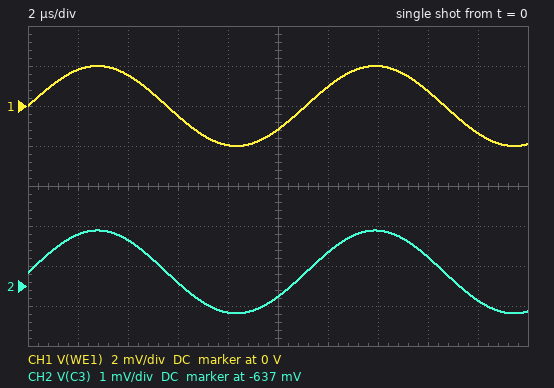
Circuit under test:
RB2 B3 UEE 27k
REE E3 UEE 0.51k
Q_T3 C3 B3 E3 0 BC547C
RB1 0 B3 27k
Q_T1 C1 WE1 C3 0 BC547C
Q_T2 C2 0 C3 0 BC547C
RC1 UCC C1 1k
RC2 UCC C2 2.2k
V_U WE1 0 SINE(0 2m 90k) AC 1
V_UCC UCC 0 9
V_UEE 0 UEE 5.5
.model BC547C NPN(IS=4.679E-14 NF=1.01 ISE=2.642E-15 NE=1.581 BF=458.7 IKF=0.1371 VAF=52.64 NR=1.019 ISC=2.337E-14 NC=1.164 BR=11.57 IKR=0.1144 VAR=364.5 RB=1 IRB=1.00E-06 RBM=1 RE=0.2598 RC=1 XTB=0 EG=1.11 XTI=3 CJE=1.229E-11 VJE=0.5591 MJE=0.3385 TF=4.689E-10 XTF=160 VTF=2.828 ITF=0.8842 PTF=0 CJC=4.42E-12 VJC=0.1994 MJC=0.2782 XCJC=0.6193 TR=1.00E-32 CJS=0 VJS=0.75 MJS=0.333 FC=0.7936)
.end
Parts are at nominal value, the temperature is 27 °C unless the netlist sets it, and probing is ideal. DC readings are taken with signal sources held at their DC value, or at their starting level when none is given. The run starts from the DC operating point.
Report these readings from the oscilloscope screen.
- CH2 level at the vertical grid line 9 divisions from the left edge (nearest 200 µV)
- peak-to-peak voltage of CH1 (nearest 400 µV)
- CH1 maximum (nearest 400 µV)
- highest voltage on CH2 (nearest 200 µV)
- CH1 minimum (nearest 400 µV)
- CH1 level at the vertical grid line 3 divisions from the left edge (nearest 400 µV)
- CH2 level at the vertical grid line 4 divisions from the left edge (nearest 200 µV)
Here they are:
-637.4 mV
4.0 mV
2.0 mV
-635.6 mV
-2.0 mV
-400 µV
-637.6 mV
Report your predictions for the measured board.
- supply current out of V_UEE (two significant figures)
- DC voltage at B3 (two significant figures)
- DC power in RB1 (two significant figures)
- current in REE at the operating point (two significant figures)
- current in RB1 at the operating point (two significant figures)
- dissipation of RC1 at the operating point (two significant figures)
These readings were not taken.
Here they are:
4.0 mA
-2.9 V
300 µW
3.9 mA
110 µA
3.9 mW
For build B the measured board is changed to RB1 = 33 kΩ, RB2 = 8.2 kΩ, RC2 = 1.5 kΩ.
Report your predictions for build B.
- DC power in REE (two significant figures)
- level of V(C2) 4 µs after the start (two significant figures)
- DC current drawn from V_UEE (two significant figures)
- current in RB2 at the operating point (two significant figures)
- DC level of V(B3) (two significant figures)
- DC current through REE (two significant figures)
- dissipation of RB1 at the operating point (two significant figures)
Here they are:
420 µW
8.3 V
1.0 mA
130 µA
-4.4 V
910 µA
590 µW
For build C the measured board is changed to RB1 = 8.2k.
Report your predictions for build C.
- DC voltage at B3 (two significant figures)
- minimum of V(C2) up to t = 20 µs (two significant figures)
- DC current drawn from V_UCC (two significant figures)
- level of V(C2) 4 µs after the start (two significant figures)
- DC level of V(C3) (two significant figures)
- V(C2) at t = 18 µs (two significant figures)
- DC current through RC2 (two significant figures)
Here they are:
-1.4 V
1.6 V
6.7 mA
2.0 V
-650 mV
1.7 V
3.3 mA
